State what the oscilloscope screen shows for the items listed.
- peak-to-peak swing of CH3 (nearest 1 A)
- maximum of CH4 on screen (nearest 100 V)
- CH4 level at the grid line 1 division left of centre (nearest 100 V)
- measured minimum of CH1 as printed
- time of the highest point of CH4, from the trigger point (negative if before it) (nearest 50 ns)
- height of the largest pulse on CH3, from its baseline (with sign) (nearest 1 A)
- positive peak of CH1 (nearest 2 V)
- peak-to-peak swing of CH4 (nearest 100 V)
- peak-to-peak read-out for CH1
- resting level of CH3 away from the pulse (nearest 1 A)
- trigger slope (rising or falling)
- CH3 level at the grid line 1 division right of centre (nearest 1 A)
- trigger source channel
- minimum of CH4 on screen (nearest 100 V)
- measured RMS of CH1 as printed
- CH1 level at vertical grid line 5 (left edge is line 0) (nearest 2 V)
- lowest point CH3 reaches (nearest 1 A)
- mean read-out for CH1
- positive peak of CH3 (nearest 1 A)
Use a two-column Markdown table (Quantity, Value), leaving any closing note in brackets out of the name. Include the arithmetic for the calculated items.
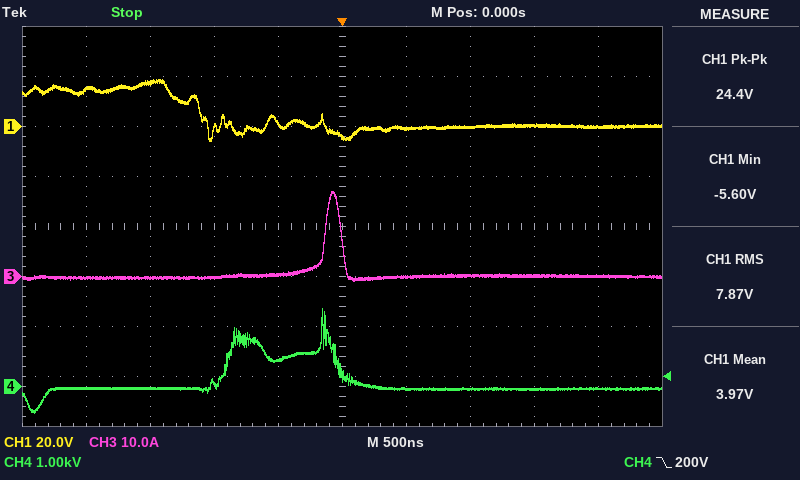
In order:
| Quantity | Value |
|---|---|
| peak-to-peak swing of CH3 | 17 A − (-1 A) = 18 A |
| maximum of CH4 on screen | 1.6 kV |
| CH4 level at the grid line 1 division left of centre | 500 V |
| measured minimum of CH1 as printed | -5.60 V |
| time of the highest point of CH4, from the trigger point (negative if before it) | -150 ns |
| height of the largest pulse on CH3, from its baseline (with sign) | 17 A − (0 A) = +17 A |
| positive peak of CH1 | 18 V |
| peak-to-peak swing of CH4 | 1.6 kV − (-500 V) = 2.1 kV |
| peak-to-peak read-out for CH1 | 24.4 V |
| resting level of CH3 away from the pulse | 0 A |
| trigger slope | falling |
| CH3 level at the grid line 1 division right of centre | 0 A |
| trigger source channel | CH4 |
| minimum of CH4 on screen | -500 V |
| measured RMS of CH1 as printed | 7.87 V |
| CH1 level at vertical grid line 5 (left edge is line 0) | -4 V |
| lowest point CH3 reaches | -1 A |
| mean read-out for CH1 | 3.97 V |
| positive peak of CH3 | 17 A |
